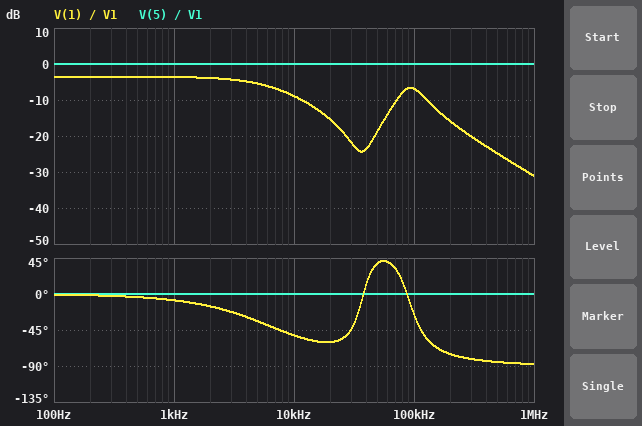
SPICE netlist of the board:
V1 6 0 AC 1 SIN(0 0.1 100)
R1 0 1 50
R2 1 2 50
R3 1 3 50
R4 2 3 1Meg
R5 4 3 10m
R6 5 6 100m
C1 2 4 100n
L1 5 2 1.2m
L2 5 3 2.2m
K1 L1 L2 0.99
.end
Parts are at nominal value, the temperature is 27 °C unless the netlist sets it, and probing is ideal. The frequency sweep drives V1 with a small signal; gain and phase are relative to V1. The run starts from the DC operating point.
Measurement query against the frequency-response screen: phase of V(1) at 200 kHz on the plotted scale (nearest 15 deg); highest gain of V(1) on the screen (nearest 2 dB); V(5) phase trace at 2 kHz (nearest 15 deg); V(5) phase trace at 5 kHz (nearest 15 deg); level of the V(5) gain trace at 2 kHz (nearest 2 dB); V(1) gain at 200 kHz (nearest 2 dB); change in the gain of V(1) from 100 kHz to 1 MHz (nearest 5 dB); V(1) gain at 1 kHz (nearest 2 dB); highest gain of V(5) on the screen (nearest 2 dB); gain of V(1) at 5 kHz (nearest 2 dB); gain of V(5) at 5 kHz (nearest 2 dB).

-75 deg
-4 dB
0 deg
0 deg
0 dB
-16 dB
-25 dB
-4 dB
0 dB
-6 dB
0 dB
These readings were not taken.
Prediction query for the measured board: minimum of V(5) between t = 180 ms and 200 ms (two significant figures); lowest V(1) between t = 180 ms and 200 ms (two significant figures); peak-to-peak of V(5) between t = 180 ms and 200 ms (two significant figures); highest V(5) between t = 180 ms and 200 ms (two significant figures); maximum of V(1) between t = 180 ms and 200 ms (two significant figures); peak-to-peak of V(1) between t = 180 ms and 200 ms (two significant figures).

-100 mV
-67 mV
200 mV
100 mV
67 mV
130 mV
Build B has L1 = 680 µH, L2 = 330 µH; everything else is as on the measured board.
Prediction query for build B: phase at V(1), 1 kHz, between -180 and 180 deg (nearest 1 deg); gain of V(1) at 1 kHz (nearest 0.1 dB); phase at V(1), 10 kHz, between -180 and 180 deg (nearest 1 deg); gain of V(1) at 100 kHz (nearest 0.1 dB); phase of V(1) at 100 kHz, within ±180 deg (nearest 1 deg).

-2 deg
-3.5 dB
-22 deg
-9.3 dB
42 deg
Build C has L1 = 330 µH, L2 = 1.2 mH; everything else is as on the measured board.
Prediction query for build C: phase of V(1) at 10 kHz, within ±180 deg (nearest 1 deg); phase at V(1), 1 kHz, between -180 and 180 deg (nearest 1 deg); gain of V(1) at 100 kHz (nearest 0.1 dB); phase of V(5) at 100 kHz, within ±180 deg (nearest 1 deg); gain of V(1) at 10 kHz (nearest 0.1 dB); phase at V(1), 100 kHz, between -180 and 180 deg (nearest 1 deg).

-29 deg
-3 deg
-4.6 dB
0 deg
-5.7 dB
15 deg
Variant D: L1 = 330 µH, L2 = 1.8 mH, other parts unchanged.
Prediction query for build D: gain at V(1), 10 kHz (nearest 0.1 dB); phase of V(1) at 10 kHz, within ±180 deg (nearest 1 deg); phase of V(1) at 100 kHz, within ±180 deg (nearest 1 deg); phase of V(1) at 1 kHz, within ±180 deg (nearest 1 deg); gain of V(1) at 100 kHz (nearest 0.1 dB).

-7.7 dB
-30 deg
8 deg
-4 deg
-4.1 dB
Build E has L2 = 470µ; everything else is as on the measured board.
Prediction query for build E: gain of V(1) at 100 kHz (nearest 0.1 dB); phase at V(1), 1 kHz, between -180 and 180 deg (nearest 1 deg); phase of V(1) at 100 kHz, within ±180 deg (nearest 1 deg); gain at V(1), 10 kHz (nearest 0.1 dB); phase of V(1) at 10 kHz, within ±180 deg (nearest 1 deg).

-5.5 dB
-4 deg
20 deg
-5.7 dB
-33 deg
